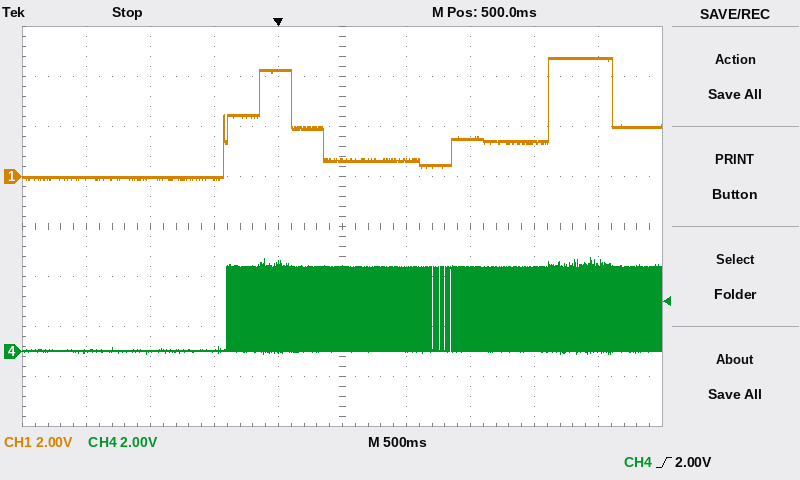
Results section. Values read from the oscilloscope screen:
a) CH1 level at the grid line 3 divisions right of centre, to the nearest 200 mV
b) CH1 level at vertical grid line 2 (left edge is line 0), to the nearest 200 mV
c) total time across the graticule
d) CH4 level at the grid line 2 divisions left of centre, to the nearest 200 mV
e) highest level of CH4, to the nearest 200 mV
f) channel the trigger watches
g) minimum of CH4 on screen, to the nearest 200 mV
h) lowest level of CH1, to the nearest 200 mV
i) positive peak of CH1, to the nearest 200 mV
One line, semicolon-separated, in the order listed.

1.4 V; 0.0 V; 5 s; 0.0 V; 3.8 V; CH4; -200 mV; -200 mV; 4.8 V
